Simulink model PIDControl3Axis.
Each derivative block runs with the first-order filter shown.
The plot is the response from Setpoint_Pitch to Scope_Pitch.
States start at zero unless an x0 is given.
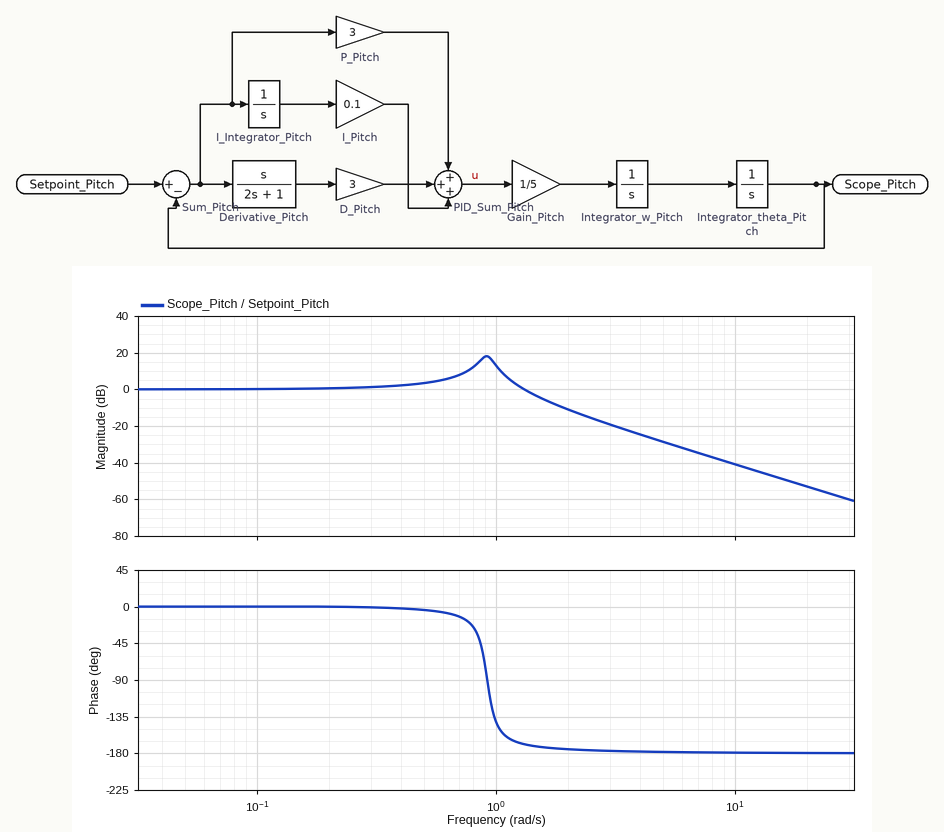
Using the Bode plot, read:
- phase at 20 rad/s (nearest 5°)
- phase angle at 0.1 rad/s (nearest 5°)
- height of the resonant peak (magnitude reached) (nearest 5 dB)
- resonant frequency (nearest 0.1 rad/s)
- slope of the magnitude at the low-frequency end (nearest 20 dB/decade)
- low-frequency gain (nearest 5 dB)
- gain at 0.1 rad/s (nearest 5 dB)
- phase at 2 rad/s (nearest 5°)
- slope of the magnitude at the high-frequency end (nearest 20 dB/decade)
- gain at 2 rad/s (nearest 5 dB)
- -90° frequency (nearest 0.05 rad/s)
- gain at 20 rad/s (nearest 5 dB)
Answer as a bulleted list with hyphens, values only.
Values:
- -180°
- 0°
- 20 dB
- 0.9 rad/s
- 0 dB/decade
- 0 dB
- 0 dB
- -175°
- -40 dB/decade
- -10 dB
- 0.90 rad/s
- -55 dB
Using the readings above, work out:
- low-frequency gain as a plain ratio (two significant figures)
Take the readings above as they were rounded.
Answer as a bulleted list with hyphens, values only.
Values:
- 1.0
